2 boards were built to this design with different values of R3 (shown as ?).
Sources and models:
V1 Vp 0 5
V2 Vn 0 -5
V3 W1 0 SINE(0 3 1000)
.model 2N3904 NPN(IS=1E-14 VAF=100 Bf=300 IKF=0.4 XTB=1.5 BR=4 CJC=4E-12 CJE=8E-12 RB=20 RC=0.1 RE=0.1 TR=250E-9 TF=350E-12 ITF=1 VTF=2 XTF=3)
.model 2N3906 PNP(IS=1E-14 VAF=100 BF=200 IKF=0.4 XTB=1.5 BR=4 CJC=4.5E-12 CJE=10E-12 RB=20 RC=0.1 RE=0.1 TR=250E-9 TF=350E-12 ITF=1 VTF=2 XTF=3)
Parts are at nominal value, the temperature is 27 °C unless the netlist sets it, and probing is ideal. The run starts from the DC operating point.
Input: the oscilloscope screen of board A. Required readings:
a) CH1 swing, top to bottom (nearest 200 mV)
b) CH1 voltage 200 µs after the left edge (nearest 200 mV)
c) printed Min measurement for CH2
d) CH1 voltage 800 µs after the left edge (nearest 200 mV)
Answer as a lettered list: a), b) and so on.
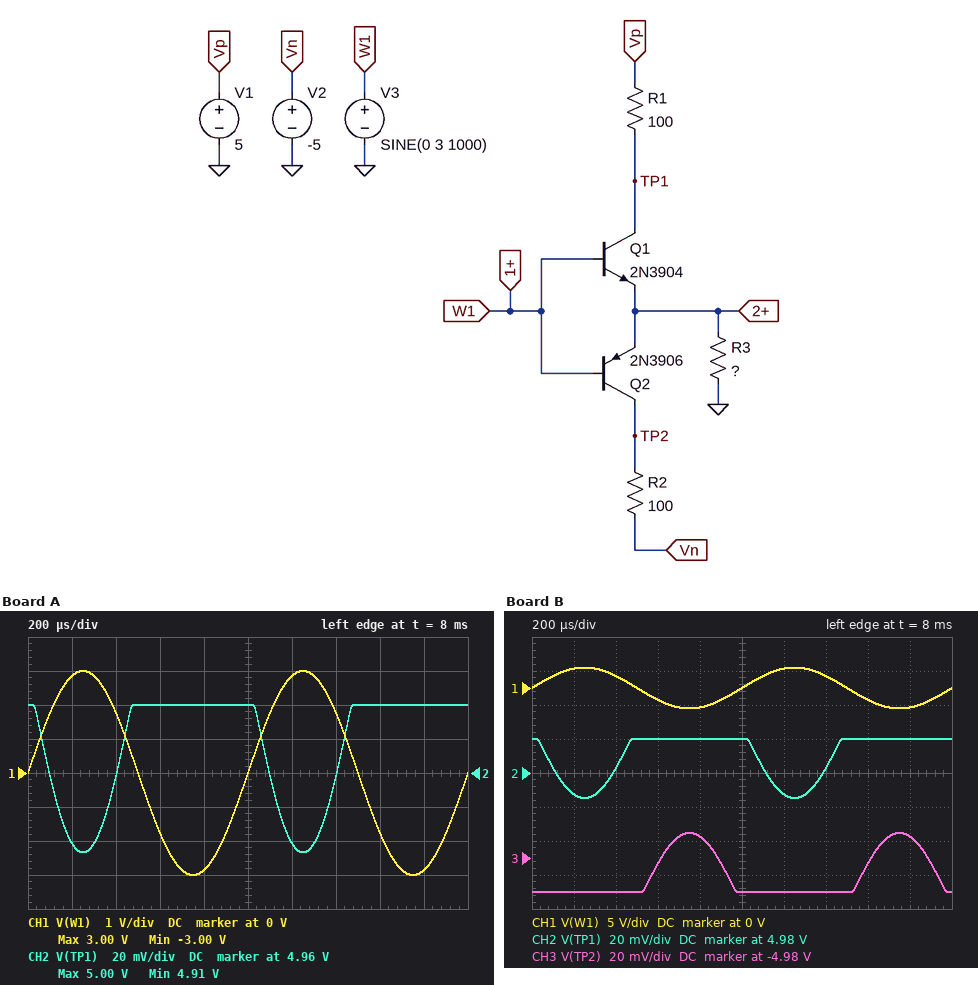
a) 6.0 V
b) 2.8 V
c) 4.91 V
d) -2.8 V
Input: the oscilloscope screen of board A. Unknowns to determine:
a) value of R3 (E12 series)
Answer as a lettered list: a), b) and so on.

a) 2.7 kΩ
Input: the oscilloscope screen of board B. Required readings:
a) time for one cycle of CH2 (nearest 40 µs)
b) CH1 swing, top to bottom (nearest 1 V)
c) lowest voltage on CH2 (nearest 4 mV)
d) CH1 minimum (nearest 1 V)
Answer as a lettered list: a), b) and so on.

a) 1.00 ms
b) 6 V
c) 4.964 V
d) -3 V
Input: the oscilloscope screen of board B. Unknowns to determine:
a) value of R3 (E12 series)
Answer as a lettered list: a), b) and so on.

a) 6.8 kΩ
